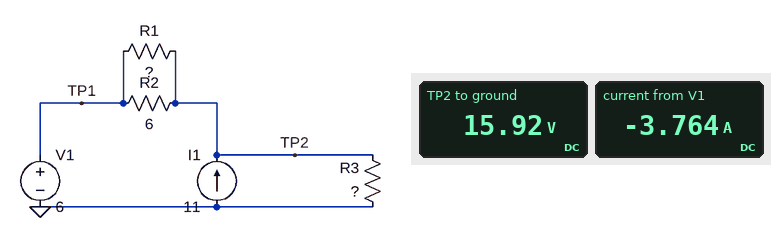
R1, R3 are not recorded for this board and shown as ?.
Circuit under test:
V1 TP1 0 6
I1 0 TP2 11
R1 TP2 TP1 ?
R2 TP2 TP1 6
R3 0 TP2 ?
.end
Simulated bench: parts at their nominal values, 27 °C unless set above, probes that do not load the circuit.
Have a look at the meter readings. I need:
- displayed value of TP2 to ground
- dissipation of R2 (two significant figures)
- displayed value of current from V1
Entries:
15.92 V
16 W
-3.764 A
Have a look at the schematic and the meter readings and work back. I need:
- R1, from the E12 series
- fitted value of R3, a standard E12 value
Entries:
4.7 Ω
2.2 Ω
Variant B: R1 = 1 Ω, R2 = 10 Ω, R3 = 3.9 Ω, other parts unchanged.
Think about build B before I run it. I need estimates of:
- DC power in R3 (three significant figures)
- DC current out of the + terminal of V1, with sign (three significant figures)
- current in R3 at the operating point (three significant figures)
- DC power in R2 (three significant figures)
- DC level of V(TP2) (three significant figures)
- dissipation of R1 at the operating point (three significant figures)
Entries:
43.2 W
-7.67 A
3.33 A
4.87 W
13.0 V
48.7 W
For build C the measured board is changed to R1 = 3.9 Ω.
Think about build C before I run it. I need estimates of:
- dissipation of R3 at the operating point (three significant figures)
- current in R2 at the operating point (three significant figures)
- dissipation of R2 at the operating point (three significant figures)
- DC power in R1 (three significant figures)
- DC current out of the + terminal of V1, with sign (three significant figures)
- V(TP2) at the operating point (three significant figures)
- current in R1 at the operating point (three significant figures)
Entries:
108 W
1.57 A
14.8 W
22.8 W
-3.99 A
15.4 V
2.42 A
